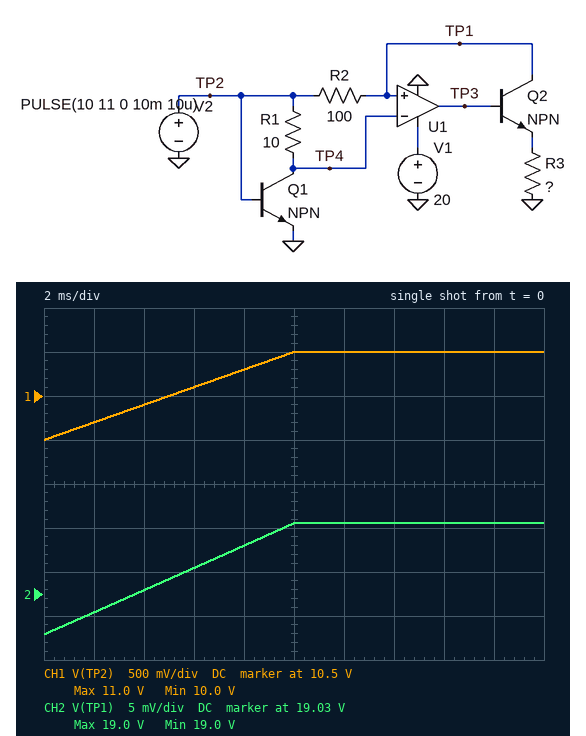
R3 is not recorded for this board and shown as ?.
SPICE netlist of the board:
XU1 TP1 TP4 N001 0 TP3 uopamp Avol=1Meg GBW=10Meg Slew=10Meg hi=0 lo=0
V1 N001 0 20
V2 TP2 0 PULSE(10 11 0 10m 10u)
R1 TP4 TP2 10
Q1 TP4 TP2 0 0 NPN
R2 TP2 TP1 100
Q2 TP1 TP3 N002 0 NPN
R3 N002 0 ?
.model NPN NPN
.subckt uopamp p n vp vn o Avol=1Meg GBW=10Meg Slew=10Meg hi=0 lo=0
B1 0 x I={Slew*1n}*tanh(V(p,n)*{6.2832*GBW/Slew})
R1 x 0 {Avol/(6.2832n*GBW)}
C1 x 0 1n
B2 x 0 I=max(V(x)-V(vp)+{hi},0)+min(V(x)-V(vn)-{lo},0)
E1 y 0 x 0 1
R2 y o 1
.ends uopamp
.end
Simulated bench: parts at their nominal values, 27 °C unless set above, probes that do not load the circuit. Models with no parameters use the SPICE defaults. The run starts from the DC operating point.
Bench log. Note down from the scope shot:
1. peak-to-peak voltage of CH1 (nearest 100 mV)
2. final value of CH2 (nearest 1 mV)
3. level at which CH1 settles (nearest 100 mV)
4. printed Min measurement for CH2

1.0 V
19.033 V
11.0 V
19.0 V
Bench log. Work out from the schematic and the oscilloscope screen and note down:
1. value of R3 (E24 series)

2.7 kΩ
